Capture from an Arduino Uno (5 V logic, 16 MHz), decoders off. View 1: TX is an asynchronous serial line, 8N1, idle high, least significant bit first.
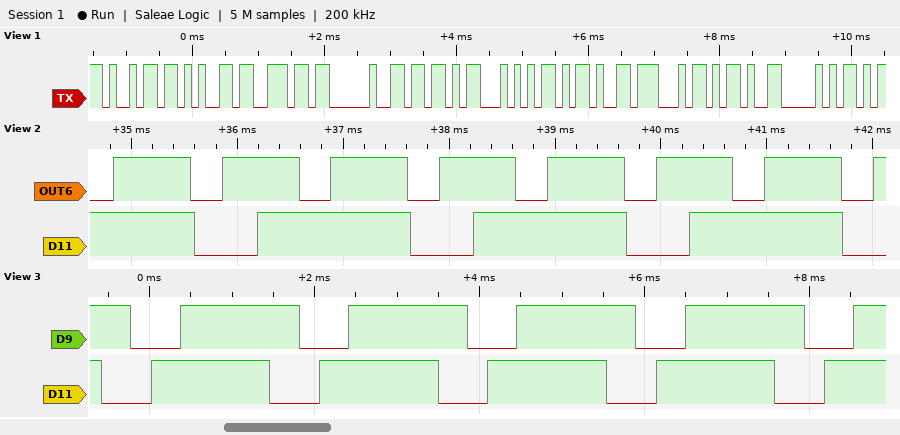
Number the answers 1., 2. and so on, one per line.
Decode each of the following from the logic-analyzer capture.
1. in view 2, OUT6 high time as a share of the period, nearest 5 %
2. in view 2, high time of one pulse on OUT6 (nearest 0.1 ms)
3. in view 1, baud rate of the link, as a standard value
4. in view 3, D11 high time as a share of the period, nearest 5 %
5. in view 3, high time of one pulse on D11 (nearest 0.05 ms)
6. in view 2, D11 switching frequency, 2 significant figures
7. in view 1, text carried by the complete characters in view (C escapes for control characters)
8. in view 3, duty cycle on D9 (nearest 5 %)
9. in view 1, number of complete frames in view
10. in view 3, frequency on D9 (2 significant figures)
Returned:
1. 70 %
2. 0.7 ms
3. 9600 baud
4. 70 %
5. 1.45 ms
6. 490 Hz
7. "ien [T-G-P"
8. 70 %
9. 10
10. 490 Hz
